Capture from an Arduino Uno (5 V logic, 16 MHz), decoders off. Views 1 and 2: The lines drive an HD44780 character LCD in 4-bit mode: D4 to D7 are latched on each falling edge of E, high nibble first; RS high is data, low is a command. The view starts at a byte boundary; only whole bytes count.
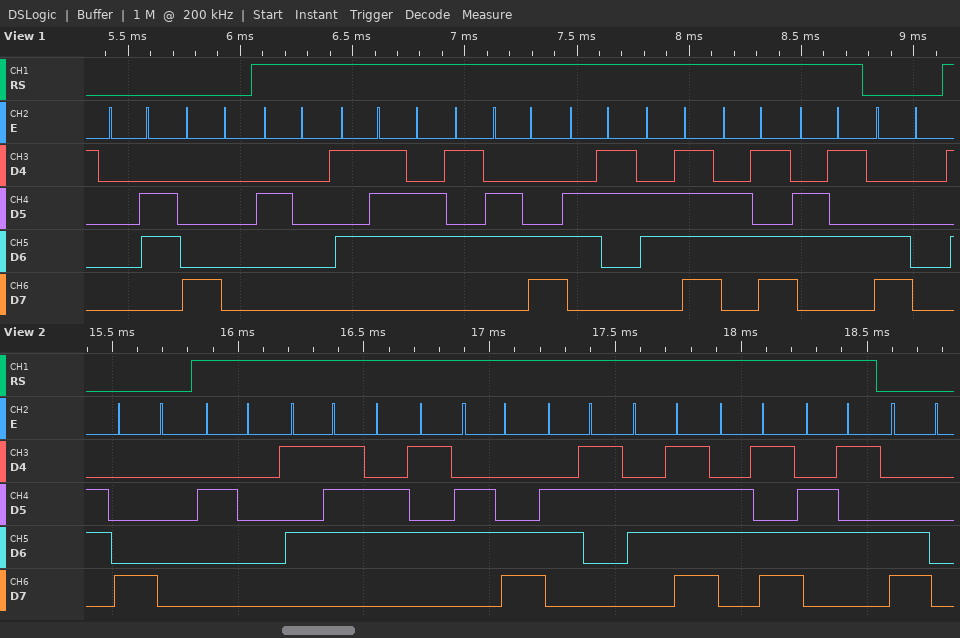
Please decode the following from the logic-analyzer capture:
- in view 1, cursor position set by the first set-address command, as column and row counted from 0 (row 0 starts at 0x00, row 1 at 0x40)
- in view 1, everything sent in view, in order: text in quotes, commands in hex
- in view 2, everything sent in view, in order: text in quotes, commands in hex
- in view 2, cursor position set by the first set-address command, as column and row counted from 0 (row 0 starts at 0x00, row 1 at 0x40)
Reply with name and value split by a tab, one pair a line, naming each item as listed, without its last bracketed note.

in view 1, cursor position set by the first set-address command, as column and row counted from 0	column 0, row 0
in view 1, everything sent in view, in order: text in quotes, commands in hex	0x06 0x80 " Welcome" 0xC0
in view 2, everything sent in view, in order: text in quotes, commands in hex	0x80 " Welcome" 0xC0
in view 2, cursor position set by the first set-address command, as column and row counted from 0	column 0, row 0
